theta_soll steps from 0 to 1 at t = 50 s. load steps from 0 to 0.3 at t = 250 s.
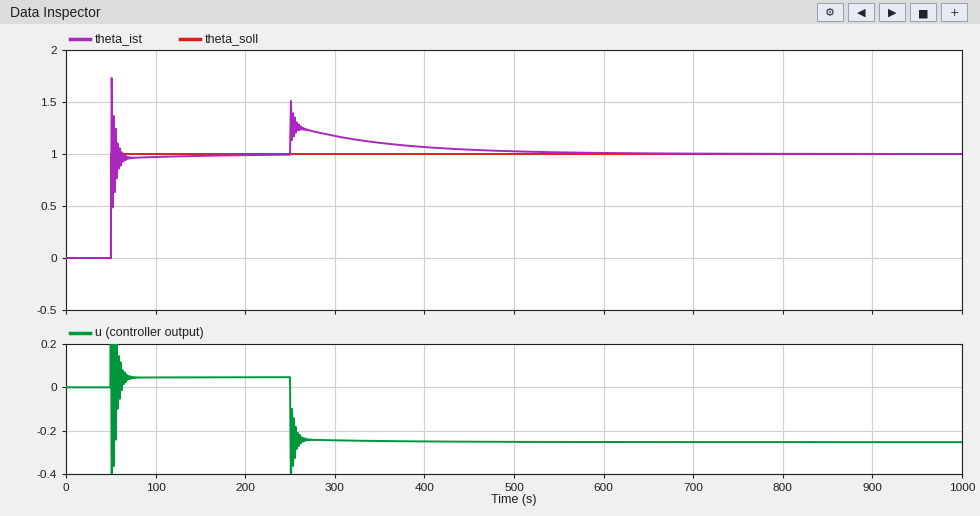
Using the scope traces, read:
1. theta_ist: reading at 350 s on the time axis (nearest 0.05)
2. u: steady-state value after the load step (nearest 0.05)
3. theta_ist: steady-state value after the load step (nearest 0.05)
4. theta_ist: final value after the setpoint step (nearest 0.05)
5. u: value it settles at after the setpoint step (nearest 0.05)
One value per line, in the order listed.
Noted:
1.10
-0.25
1.00
1.00
0.05
